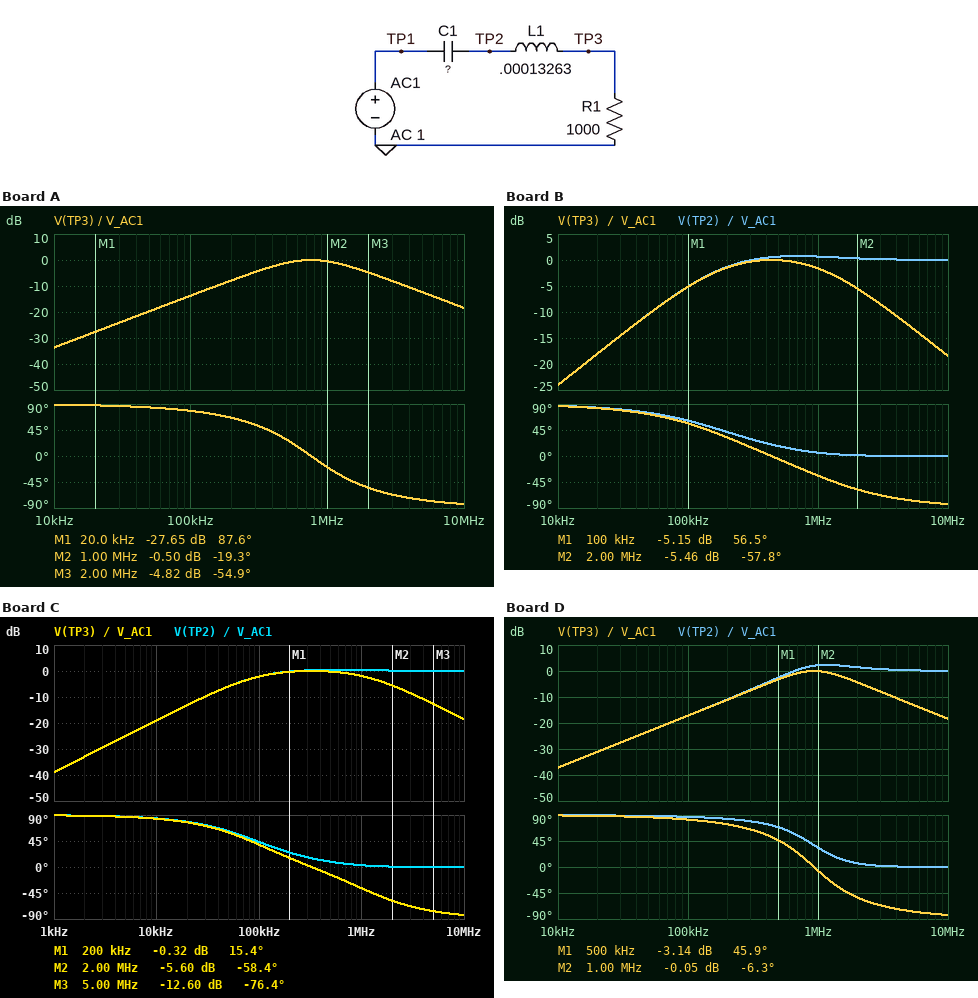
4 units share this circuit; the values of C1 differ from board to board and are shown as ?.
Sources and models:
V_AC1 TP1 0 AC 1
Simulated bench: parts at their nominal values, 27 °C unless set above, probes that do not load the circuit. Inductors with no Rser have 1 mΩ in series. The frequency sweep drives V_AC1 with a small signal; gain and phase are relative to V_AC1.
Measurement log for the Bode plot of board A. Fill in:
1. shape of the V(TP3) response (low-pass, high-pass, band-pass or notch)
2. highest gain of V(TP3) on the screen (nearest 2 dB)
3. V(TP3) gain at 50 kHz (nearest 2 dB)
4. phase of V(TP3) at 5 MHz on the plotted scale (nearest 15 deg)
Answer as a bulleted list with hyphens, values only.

- band-pass
- 0 dB
- -20 dB
- -75 deg
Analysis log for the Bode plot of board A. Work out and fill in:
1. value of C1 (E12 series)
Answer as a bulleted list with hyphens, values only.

- 330 pF
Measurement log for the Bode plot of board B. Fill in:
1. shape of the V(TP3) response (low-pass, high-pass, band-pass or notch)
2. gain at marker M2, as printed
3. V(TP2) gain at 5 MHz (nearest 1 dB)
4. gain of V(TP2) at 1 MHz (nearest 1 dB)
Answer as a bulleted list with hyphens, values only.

- band-pass
- -5.46 dB
- 0 dB
- 1 dB
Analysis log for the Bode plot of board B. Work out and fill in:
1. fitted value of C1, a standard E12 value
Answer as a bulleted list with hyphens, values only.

- 1 nF
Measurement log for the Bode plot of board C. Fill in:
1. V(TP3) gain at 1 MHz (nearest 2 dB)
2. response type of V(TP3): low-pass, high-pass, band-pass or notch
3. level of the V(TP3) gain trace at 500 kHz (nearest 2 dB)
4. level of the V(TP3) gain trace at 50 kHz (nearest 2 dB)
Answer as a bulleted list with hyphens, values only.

- -2 dB
- band-pass
- 0 dB
- -6 dB
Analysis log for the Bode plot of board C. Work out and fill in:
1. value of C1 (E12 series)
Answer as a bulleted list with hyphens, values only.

- 1.8 nF
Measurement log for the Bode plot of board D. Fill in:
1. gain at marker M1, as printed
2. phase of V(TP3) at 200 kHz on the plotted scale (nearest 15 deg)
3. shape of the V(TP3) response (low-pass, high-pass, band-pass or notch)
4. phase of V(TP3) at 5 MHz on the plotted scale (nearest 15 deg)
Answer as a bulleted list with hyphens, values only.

- -3.14 dB
- 75 deg
- band-pass
- -75 deg
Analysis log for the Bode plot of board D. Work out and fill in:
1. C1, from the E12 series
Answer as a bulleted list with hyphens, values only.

- 220 pF
